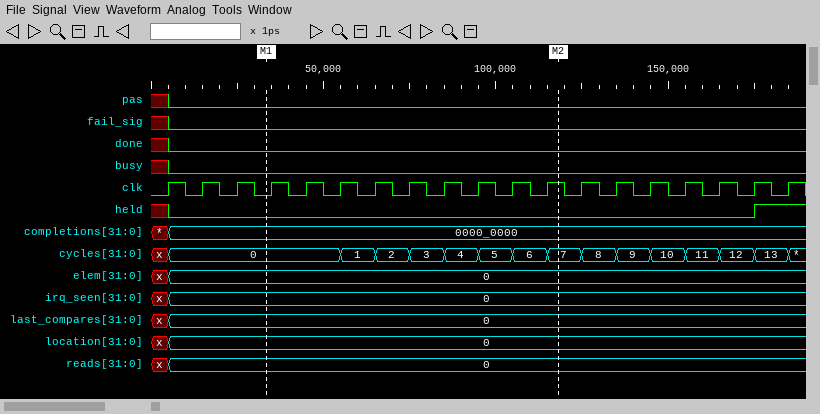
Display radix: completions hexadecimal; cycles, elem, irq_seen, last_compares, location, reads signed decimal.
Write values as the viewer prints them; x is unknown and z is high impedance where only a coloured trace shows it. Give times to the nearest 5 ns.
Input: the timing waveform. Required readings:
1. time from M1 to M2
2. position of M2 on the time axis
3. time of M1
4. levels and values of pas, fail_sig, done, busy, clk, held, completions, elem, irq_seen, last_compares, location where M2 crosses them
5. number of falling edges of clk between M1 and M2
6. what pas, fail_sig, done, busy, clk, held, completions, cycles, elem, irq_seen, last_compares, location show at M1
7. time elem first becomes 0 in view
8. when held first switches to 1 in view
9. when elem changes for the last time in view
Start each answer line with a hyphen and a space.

- 85 ns
- 120 ns
- 35 ns
- pas=0, fail_sig=0, done=0, busy=0, clk=1, held=0, completions=0000_0000, elem=0, irq_seen=0, last_compares=0, location=0
- 8
- pas=0, fail_sig=0, done=0, busy=0, clk=0, held=0, completions=0000_0000, cycles=0, elem=0, irq_seen=0, last_compares=0, location=0
- 5 ns
- 175 ns
- 5 ns
